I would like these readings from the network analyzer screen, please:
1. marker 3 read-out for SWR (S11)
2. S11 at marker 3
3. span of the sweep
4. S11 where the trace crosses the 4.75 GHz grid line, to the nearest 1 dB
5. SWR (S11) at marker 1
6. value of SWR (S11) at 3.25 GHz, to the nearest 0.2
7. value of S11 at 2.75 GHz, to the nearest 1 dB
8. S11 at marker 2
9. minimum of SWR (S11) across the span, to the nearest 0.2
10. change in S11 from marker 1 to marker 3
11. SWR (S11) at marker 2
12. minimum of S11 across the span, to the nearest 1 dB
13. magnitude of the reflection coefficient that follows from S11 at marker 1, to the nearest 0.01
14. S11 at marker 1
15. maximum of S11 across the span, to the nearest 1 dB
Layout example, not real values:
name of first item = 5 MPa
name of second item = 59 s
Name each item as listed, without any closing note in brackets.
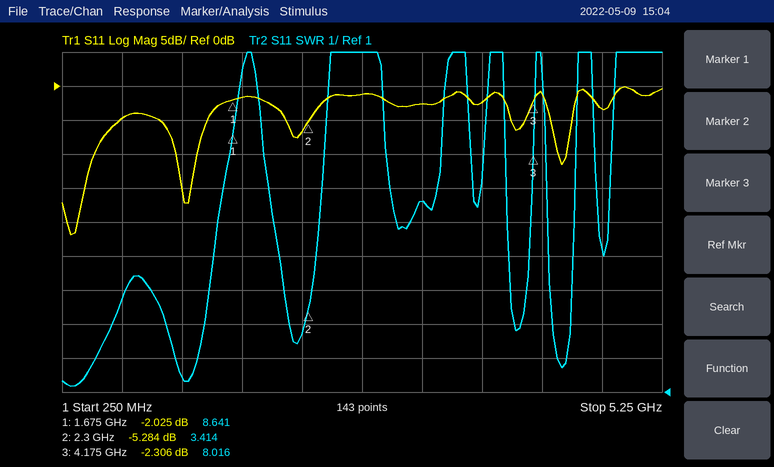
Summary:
marker 3 read-out for SWR = 8.016
S11 at marker 3 = -2.306 dB
span of the sweep = 5 GHz
S11 where the trace crosses the 4.75 GHz grid line, to the nearest 1 dB = -3 dB
SWR (S11) at marker 1 = 8.641
value of SWR (S11) at 3.25 GHz, to the nearest 0.2 = 6.6
value of S11 at 2.75 GHz, to the nearest 1 dB = -1 dB
S11 at marker 2 = -5.284 dB
minimum of SWR (S11) across the span, to the nearest 0.2 = 1.2
change in S11 from marker 1 to marker 3 = -0.281 dB
SWR (S11) at marker 2 = 3.414
minimum of S11 across the span, to the nearest 1 dB = -22 dB
magnitude of the reflection coefficient that follows from S11 at marker 1, to the nearest 0.01 = 0.79
S11 at marker 1 = -2.025 dB
maximum of S11 across the span, to the nearest 1 dB = 0 dB
